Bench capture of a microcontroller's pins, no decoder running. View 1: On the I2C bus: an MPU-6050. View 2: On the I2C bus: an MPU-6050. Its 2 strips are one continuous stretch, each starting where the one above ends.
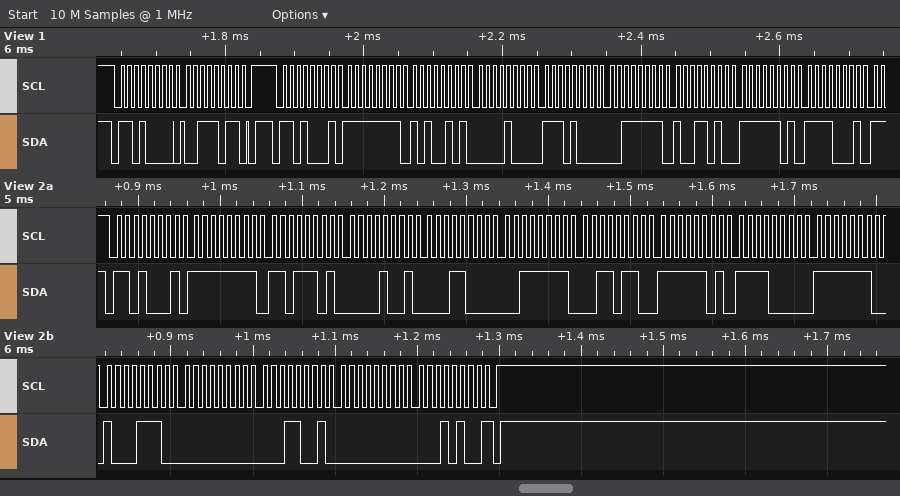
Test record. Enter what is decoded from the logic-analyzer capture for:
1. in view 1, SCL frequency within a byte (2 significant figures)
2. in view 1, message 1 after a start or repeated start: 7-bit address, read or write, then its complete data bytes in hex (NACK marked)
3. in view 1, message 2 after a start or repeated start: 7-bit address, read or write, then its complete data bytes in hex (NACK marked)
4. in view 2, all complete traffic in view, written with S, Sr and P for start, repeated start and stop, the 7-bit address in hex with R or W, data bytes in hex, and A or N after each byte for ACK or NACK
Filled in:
100 kHz
0x68 write: 3B
0x68 read: FF A5 08 E8 3F 9A FD F1
S 68R A FF A DD A 09 A 18 A 3F A 36 A FD A F0 A FE A 8E A 00 A 19 A 00 A 14 N P
